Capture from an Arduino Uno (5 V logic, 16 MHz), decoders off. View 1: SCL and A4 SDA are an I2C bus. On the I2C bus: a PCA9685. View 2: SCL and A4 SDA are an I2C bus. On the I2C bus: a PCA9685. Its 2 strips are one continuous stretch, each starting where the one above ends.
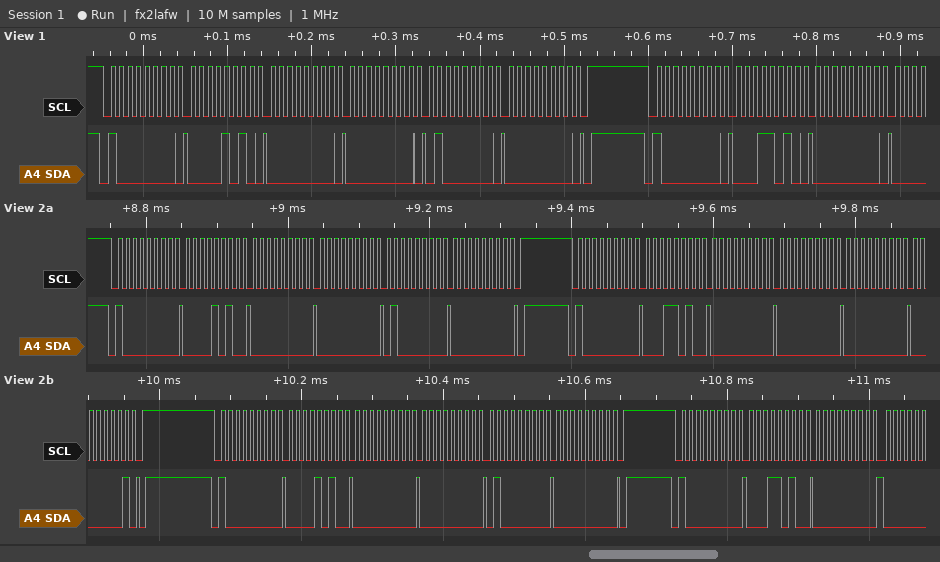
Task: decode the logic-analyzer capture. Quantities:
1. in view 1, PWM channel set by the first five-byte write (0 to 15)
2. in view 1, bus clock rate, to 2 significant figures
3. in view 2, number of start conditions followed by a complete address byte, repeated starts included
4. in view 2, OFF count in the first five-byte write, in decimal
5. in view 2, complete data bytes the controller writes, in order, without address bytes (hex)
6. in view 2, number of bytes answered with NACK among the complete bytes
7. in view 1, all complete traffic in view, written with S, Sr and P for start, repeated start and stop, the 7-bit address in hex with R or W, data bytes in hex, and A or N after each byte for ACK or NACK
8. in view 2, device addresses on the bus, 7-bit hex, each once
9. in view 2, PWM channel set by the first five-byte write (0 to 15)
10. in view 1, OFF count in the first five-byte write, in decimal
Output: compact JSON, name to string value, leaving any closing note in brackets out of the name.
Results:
{"in view 1, PWM channel set by the first five-byte write": "1", "in view 1, bus clock rate, to 2 significant figures": "100 kHz", "in view 2, number of start conditions followed by a complete address byte, repeated starts included": "4", "in view 2, OFF count in the first five-byte write, in decimal": "64", "in view 2, complete data bytes the controller writes, in order, without address bytes": "0A 00 00 40 00 1A 00 00 00 01 0A 00 00 40 00 1A 00", "in view 2, number of bytes answered with NACK among the complete bytes": "0", "in view 1, all complete traffic in view, written with S, Sr and P for start, repeated start and stop, the 7-bit address in hex with R or W, data bytes in hex, and A or N after each byte for ACK or NACK": "S 40W A 0A A 00 A 00 A 40 A 00 A P S 40W A 1A A 00 A", "in view 2, device addresses on the bus, 7-bit hex, each once": "0x40", "in view 2, PWM channel set by the first five-byte write": "1", "in view 1, OFF count in the first five-byte write, in decimal": "64"}
